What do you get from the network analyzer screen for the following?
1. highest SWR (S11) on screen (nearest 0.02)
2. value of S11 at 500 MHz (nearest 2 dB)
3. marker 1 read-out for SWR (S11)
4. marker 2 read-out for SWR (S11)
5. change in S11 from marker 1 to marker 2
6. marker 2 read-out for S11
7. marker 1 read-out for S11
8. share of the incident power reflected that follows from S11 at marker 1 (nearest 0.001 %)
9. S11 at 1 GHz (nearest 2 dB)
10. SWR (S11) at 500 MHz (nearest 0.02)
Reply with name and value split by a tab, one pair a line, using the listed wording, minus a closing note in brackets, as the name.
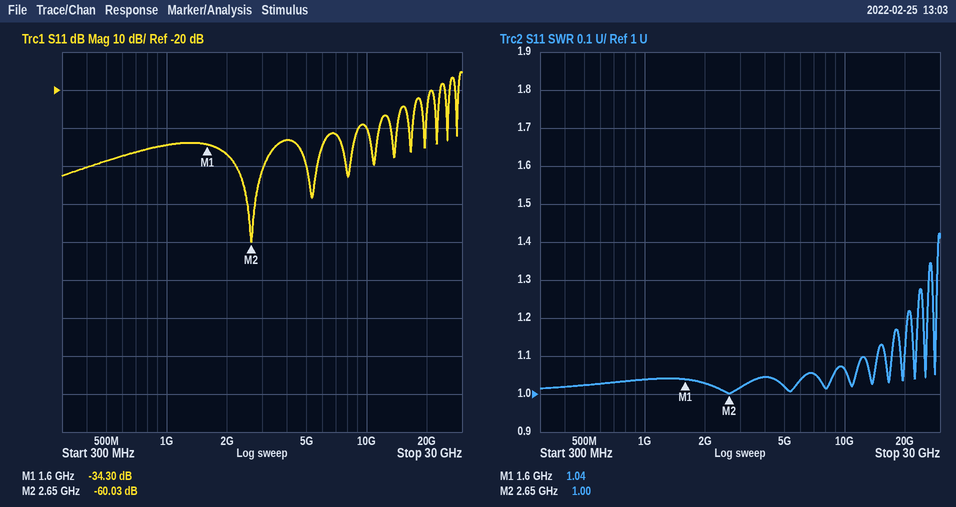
highest SWR (S11) on screen	1.42
value of S11 at 500 MHz	-38 dB
marker 1 read-out for SWR	1.04
marker 2 read-out for SWR	1.00
change in S11 from marker 1 to marker 2	-25.73 dB
marker 2 read-out for S11	-60.03 dB
marker 1 read-out for S11	-34.30 dB
share of the incident power reflected that follows from S11 at marker 1	0.037 %
S11 at 1 GHz	-34 dB
SWR (S11) at 500 MHz	1.02
